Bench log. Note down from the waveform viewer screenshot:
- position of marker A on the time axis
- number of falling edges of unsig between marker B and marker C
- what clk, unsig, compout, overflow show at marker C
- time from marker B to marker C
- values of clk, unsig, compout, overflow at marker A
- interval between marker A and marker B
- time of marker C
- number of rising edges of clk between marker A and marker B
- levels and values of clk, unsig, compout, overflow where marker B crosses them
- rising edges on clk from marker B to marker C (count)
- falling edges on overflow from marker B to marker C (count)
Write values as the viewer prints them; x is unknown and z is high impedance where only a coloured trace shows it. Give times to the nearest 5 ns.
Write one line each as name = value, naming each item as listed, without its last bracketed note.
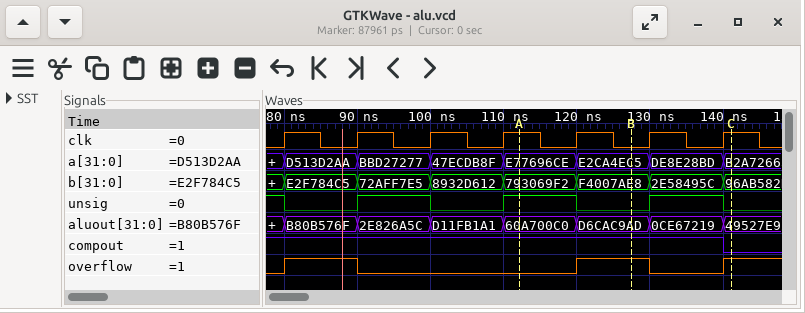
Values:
position of marker A on the time axis = 110 ns
number of falling edges of unsig between marker B and marker C = 1
what clk, unsig, compout, overflow show at marker C = clk=1, unsig=0, compout=0, overflow=1
time from marker B to marker C = 15 ns
values of clk, unsig, compout, overflow at marker A = clk=1, unsig=1, compout=1, overflow=0
interval between marker A and marker B = 15 ns
time of marker C = 140 ns
number of rising edges of clk between marker A and marker B = 1
levels and values of clk, unsig, compout, overflow where marker B crosses them = clk=0, unsig=0, compout=1, overflow=1
rising edges on clk from marker B to marker C = 2
falling edges on overflow from marker B to marker C = 1
